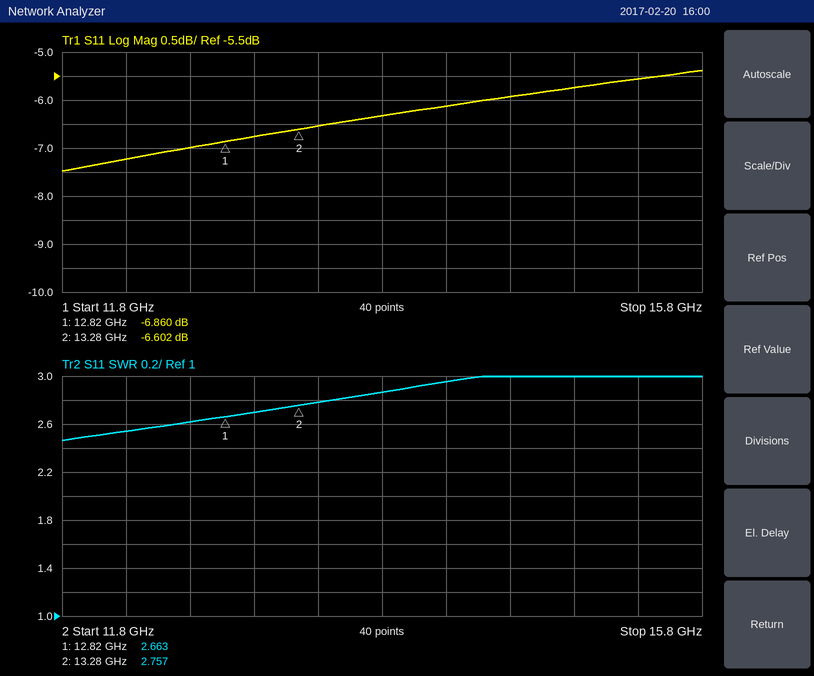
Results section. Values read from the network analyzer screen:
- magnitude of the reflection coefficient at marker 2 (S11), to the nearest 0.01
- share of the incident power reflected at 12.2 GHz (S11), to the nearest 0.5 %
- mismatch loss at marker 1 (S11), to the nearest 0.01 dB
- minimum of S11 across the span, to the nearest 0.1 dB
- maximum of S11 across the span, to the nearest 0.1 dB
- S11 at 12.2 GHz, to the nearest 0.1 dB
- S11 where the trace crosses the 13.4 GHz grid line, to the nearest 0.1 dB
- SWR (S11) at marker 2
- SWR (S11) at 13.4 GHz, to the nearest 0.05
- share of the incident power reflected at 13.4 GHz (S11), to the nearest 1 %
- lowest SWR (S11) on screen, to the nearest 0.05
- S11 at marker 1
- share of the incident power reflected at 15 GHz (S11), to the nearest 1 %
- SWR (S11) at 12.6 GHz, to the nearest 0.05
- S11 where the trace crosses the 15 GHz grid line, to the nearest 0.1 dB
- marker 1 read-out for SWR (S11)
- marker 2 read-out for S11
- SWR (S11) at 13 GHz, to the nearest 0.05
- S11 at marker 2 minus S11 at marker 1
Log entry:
0.47
19.0 %
1.00 dB
-7.5 dB
-5.4 dB
-7.2 dB
-6.5 dB
2.757
2.80
22 %
2.45
-6.860 dB
27 %
2.60
-5.7 dB
2.663
-6.602 dB
2.70
0.258 dB
